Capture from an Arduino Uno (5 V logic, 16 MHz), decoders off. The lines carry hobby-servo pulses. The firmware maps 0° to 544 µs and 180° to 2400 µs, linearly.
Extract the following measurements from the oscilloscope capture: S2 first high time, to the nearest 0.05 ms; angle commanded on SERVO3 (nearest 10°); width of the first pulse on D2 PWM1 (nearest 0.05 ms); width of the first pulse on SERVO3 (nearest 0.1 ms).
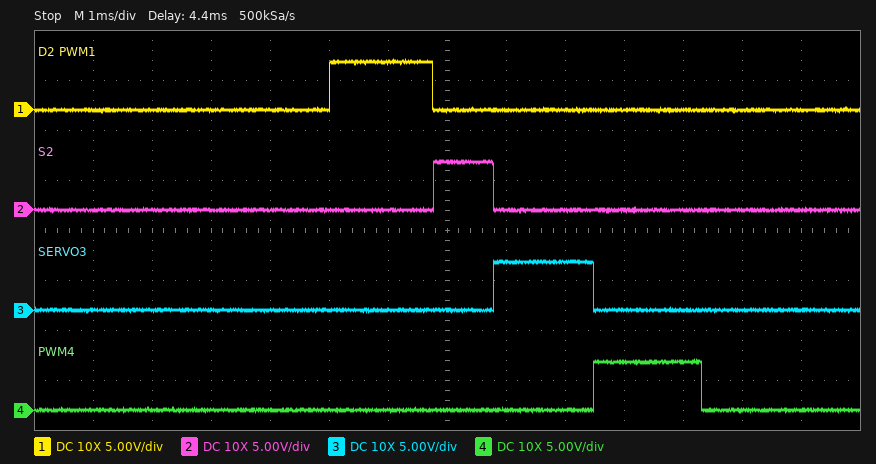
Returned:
1.00 ms
110°
1.75 ms
1.7 ms
